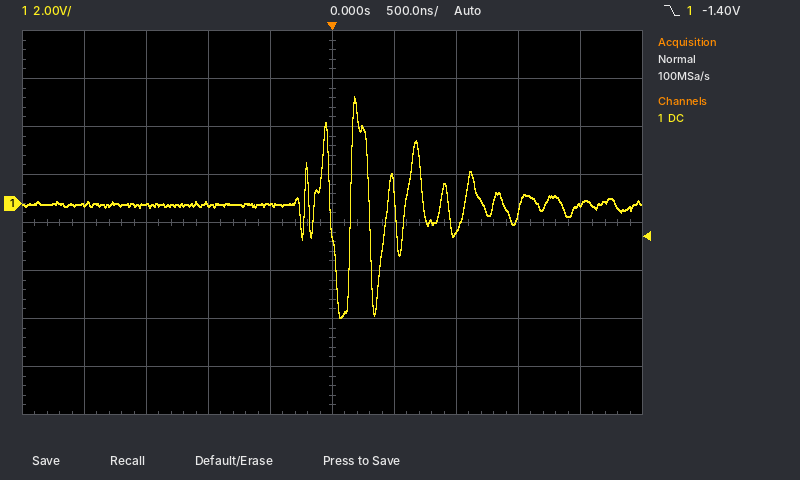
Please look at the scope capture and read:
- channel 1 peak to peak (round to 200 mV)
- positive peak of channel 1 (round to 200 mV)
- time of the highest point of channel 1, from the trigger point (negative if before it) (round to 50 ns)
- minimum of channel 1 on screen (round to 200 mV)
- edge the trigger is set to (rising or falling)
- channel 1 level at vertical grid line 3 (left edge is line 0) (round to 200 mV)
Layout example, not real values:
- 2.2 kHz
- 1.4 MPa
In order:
- 9.2 V
- 4.4 V
- +200 ns
- -4.8 V
- falling
- 0.0 V
